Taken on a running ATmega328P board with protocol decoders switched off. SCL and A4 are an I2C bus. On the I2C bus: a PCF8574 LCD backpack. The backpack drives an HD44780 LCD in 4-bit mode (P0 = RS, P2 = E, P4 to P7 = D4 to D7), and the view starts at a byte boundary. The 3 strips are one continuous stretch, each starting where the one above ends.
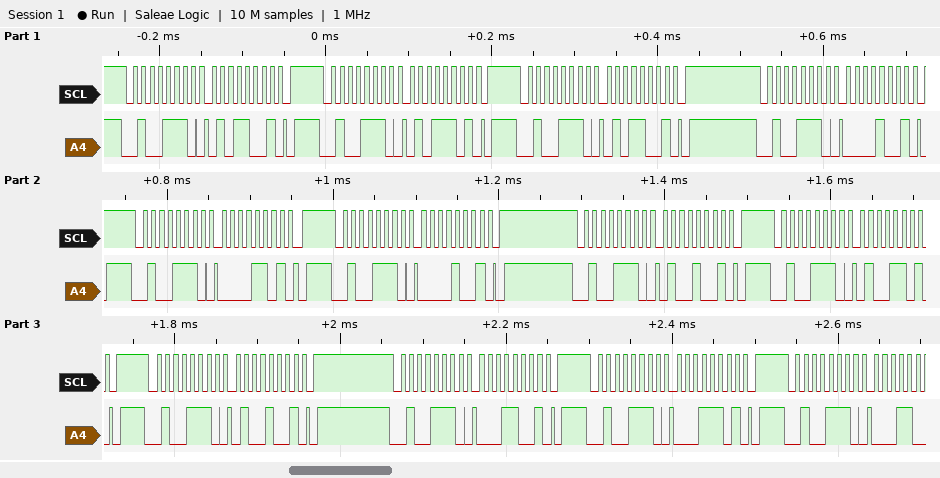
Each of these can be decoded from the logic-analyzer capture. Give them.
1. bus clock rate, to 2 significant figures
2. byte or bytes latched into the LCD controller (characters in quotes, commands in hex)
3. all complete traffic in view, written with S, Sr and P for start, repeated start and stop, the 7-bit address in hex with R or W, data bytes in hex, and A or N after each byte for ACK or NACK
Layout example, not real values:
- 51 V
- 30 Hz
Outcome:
- 100 kHz
- 'P'
- S 27W A 59 A P S 27W A 5D A P S 27W A 59 A P S 27W A 09 A P S 27W A 0D A P S 27W A 09 A P S 27W A 49 A P S 27W A 4D A P S 27W A 49 A P S 27W A 19 A P S 27W A 1D A P S 27W A
